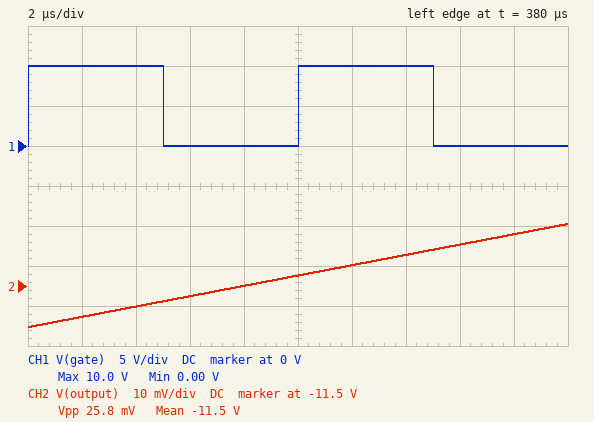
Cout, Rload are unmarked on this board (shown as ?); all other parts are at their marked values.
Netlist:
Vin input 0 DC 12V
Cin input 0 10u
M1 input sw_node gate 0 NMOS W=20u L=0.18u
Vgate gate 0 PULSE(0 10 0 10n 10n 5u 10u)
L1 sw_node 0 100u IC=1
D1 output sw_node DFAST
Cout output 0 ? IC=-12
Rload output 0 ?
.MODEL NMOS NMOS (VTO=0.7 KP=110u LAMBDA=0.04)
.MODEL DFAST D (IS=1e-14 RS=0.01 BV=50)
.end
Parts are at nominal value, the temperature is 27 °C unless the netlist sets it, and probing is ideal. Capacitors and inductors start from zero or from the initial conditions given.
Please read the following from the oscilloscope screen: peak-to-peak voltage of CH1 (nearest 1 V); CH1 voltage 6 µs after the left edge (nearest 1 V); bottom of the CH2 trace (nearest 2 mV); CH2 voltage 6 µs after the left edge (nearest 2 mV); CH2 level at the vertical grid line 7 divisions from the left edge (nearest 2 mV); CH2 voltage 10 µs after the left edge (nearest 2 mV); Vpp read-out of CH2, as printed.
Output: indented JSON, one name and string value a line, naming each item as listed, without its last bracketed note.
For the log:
{
  "peak-to-peak voltage of CH1": "10 V",
  "CH1 voltage 6 µs after the left edge": "0 V",
  "bottom of the CH2 trace": "-11.510 V",
  "CH2 voltage 6 µs after the left edge": "-11.502 V",
  "CH2 level at the vertical grid line 7 divisions from the left edge": "-11.492 V",
  "CH2 voltage 10 µs after the left edge": "-11.498 V",
  "Vpp read-out of CH2, as printed": "25.8 mV"
}
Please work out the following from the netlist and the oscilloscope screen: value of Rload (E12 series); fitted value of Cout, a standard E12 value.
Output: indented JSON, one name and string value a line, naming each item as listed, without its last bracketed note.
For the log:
{
  "value of Rload": "27 Ω",
  "fitted value of Cout, a standard E12 value": "330 µF"
}
